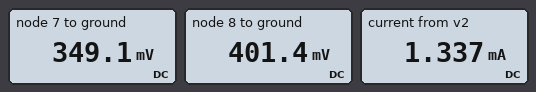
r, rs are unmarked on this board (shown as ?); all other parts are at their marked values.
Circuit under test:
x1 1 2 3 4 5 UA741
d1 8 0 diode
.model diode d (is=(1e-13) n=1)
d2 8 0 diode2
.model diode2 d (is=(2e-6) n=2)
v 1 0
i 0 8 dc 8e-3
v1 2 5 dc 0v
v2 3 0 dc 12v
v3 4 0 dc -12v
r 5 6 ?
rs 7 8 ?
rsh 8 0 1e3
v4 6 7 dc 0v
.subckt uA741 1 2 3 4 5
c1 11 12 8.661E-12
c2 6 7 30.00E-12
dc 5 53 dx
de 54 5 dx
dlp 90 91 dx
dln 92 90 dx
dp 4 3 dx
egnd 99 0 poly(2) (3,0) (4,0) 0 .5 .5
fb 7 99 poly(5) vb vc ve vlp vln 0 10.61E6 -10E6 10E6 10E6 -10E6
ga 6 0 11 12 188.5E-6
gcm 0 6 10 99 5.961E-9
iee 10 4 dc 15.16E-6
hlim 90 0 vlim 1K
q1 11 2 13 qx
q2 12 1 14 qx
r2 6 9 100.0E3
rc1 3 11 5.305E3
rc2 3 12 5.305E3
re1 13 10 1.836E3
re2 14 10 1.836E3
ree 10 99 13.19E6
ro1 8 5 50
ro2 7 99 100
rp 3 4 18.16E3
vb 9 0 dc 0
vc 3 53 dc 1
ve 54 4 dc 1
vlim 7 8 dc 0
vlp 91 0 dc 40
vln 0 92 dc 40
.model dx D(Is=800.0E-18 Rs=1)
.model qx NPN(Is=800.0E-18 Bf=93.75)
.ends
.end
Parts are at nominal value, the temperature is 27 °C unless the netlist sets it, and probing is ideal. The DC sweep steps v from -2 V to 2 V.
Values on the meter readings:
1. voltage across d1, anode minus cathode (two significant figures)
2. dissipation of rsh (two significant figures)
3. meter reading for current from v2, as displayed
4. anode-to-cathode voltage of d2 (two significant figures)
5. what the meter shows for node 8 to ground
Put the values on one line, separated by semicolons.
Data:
400 mV; 160 µW; 1.337 mA; 400 mV; 401.4 mV
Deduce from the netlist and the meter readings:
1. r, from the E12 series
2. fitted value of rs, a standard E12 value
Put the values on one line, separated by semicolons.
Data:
120 Ω; 18 Ω
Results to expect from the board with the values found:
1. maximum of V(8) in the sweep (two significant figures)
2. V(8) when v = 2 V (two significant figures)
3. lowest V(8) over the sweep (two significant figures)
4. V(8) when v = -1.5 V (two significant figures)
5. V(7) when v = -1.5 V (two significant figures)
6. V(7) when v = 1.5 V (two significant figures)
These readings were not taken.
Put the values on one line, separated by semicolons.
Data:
470 mV; 470 mV; -790 mV; -350 mV; -500 mV; 600 mV
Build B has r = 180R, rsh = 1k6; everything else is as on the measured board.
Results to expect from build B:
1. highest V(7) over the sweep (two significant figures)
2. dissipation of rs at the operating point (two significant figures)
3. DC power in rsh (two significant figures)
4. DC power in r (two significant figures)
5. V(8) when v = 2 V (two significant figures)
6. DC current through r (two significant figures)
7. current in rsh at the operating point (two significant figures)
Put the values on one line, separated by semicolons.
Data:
600 mV; 78 µW; 110 µW; 780 µW; 460 mV; 2.1 mA; 260 µA
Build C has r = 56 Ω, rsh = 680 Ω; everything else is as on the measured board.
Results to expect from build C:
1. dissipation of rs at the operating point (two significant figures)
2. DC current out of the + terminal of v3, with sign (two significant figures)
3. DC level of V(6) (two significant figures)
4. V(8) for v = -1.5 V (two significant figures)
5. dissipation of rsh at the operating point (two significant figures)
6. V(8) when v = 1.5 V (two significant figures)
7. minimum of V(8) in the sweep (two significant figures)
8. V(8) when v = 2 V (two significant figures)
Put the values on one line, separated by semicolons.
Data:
450 µW; -1.3 mA; 280 mV; -820 mV; 200 µW; 480 mV; -1.3 V; 490 mV
